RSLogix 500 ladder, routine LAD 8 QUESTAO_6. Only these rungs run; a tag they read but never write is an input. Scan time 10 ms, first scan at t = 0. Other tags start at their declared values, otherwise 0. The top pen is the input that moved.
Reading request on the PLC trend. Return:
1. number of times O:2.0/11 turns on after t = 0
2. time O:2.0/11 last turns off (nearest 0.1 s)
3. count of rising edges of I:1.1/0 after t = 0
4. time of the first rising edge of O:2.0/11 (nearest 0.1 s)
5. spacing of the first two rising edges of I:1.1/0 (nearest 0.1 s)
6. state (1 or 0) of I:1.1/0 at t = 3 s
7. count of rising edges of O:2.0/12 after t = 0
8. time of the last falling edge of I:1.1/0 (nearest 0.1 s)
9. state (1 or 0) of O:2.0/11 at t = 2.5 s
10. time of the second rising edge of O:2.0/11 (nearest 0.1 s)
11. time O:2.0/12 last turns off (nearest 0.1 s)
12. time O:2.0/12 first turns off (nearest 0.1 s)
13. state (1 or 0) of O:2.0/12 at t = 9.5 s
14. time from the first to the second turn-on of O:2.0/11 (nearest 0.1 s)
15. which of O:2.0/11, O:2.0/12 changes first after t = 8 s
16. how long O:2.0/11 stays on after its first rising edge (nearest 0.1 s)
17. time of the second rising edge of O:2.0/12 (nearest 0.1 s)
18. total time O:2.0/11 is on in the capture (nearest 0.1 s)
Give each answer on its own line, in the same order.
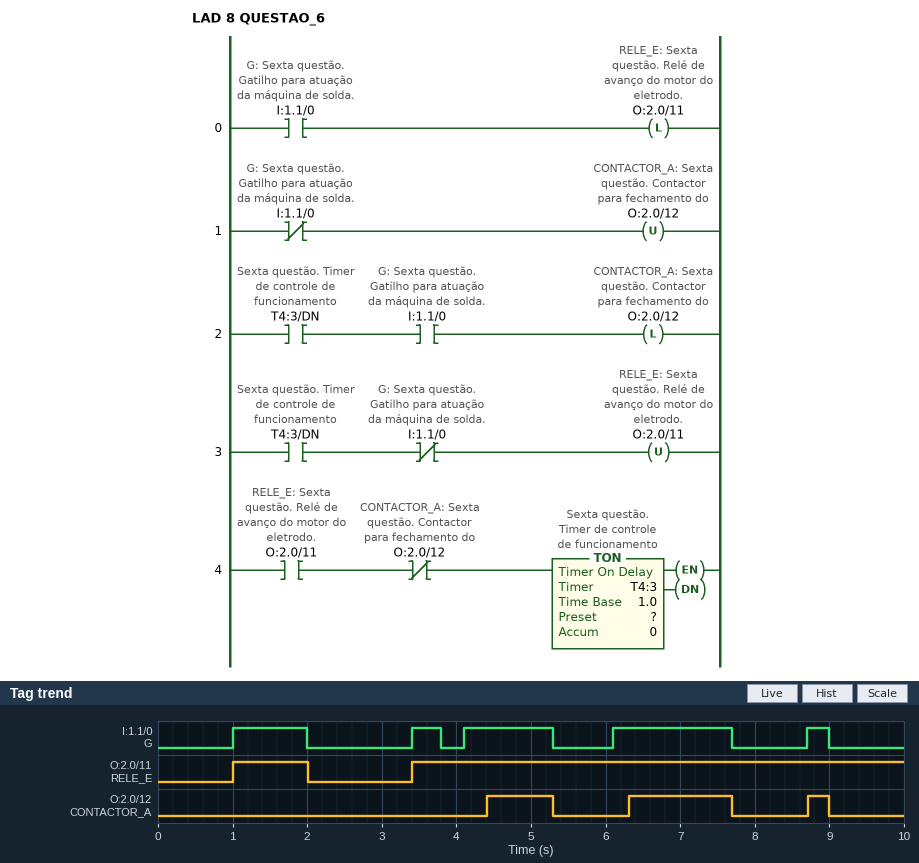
2
2.0 s
5
1.0 s
2.4 s
0
3
9.0 s
0
3.4 s
9.0 s
5.3 s
0
2.4 s
O:2.0/12
1.0 s
6.3 s
7.6 s
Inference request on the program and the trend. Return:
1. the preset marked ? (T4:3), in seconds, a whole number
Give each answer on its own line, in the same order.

1 s
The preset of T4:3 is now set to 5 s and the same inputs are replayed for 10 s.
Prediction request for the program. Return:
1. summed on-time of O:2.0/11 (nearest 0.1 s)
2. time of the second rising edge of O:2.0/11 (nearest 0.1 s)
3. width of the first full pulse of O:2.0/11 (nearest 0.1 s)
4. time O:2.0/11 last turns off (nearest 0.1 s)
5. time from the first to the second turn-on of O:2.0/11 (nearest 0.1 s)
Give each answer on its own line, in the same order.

8.9 s
6.1 s
5.0 s
6.0 s
5.1 s
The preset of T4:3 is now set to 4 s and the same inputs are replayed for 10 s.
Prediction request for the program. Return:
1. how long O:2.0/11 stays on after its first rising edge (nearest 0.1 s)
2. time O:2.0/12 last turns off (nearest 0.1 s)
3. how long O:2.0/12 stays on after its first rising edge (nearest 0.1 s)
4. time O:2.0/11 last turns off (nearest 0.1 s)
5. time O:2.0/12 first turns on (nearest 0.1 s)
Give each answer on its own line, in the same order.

8.3 s
5.3 s
0.3 s
9.3 s
5.0 s
